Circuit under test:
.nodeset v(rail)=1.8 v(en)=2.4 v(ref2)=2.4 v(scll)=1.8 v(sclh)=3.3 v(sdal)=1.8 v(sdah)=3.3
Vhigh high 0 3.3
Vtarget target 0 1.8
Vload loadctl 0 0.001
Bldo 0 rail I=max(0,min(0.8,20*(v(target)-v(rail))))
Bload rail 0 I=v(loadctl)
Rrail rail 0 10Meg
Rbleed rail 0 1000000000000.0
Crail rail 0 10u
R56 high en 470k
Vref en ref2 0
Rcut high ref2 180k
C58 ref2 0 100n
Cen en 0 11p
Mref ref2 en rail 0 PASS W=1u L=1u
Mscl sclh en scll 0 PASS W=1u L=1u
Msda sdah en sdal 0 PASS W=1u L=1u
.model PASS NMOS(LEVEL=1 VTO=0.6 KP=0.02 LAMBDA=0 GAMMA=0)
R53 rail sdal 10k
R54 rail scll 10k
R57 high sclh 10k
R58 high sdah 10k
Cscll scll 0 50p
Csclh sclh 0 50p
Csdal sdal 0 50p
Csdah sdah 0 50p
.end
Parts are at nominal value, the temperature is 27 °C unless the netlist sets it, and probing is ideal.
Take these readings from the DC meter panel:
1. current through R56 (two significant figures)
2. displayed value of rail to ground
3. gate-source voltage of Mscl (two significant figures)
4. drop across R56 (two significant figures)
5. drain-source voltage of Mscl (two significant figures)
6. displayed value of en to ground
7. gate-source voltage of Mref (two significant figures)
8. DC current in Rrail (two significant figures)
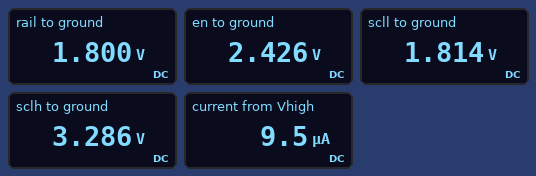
1.9 µA
1.800 V
610 mV
870 mV
1.5 V
2.426 V
630 mV
180 nA
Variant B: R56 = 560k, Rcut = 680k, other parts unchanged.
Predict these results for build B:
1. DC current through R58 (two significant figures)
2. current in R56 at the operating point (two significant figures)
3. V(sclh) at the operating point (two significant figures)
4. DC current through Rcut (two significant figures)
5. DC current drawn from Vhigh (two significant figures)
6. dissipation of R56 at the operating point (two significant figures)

800 nA
1.6 µA
3.3 V
1.3 µA
4.5 µA
1.4 µW
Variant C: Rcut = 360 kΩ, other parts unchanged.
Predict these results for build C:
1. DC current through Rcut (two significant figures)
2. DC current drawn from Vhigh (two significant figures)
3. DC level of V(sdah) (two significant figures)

2.4 µA
6.4 µA
3.3 V
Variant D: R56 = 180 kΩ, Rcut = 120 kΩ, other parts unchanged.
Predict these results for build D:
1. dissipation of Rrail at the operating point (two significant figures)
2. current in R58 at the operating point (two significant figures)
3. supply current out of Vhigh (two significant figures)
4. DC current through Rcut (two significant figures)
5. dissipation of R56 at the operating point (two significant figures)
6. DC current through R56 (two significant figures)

320 nW
2.0 µA
16 µA
7.2 µA
4.2 µW
4.8 µA
